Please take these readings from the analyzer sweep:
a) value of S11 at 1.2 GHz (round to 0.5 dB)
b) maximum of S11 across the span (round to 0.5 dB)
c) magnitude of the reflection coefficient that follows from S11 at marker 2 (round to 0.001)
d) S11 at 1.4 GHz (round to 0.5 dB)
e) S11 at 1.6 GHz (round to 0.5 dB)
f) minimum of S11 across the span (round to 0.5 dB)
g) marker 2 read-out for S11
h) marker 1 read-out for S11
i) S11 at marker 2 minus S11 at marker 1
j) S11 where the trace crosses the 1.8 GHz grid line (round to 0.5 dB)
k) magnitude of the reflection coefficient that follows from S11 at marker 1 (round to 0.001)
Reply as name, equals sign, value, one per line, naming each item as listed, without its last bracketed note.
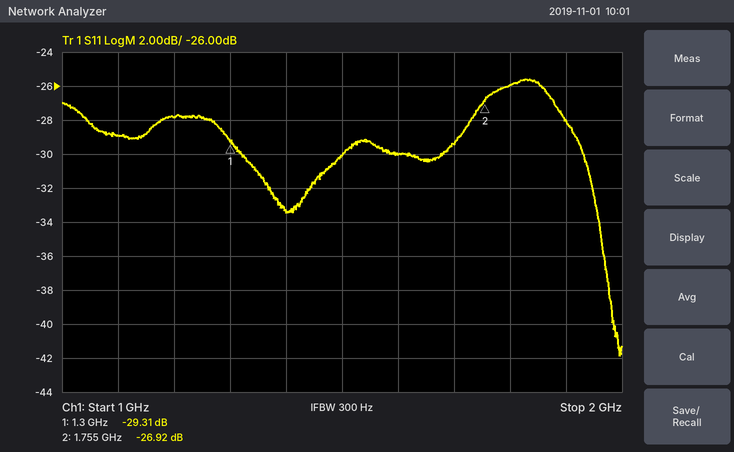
value of S11 at 1.2 GHz = -28.0 dB
maximum of S11 across the span = -25.5 dB
magnitude of the reflection coefficient that follows from S11 at marker 2 = 0.045
S11 at 1.4 GHz = -33.5 dB
S11 at 1.6 GHz = -30.0 dB
minimum of S11 across the span = -42.0 dB
marker 2 read-out for S11 = -26.92 dB
marker 1 read-out for S11 = -29.31 dB
S11 at marker 2 minus S11 at marker 1 = 2.39 dB
S11 where the trace crosses the 1.8 GHz grid line = -26.0 dB
magnitude of the reflection coefficient that follows from S11 at marker 1 = 0.034
